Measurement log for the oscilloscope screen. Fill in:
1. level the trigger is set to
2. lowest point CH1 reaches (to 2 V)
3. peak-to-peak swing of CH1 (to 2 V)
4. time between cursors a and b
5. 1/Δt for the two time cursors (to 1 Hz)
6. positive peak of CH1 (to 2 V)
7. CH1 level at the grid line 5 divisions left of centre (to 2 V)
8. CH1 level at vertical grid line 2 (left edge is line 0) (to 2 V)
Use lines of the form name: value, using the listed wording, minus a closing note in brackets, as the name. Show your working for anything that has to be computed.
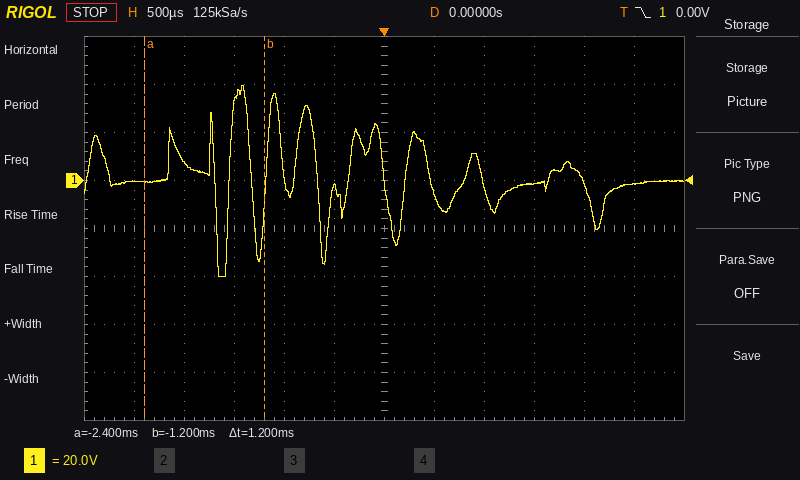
level the trigger is set to: 0.00 V
lowest point CH1 reaches: -40 V
peak-to-peak swing of CH1: 40 V − (-40 V) = 80 V
time between cursors a and b: 1.2 ms
1/Δt for the two time cursors: 1 / 1.2 ms ≈ 833 Hz
positive peak of CH1: 40 V
CH1 level at the grid line 5 divisions left of centre: 0 V
CH1 level at vertical grid line 2 (left edge is line 0): 8 V
